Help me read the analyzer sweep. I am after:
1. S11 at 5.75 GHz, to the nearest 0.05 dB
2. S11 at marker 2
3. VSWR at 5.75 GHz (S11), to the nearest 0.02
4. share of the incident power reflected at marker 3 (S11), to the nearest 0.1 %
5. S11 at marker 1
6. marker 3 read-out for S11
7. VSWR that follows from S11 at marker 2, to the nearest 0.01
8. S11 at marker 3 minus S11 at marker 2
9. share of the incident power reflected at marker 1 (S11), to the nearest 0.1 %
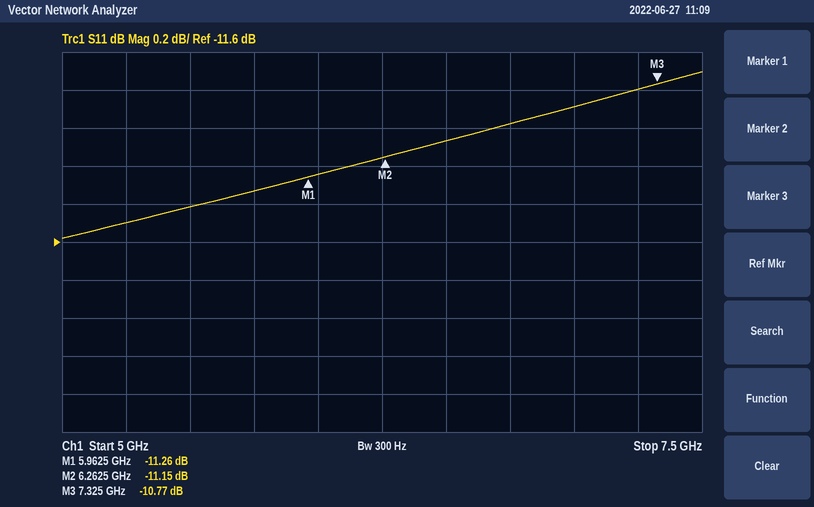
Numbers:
-11.35 dB
-11.15 dB
1.74
8.4 %
-11.26 dB
-10.77 dB
1.77
0.38 dB
7.5 %
